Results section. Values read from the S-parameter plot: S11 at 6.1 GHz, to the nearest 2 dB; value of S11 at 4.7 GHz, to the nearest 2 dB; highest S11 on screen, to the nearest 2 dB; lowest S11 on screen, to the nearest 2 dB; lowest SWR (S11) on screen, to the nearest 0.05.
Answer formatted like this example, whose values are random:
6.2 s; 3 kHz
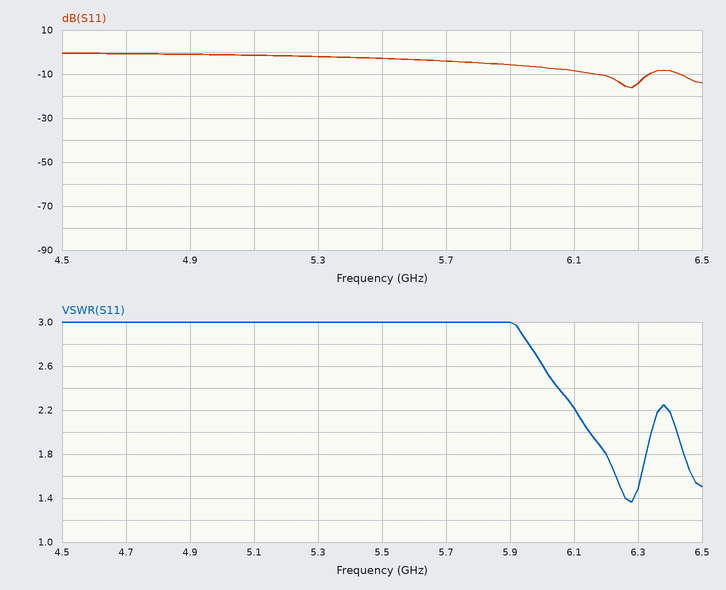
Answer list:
-8 dB; 0 dB; 0 dB; -16 dB; 1.35
